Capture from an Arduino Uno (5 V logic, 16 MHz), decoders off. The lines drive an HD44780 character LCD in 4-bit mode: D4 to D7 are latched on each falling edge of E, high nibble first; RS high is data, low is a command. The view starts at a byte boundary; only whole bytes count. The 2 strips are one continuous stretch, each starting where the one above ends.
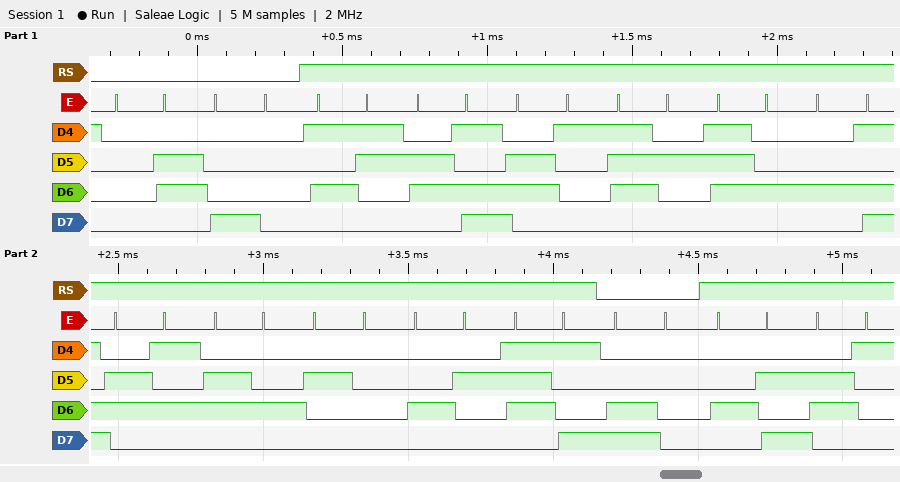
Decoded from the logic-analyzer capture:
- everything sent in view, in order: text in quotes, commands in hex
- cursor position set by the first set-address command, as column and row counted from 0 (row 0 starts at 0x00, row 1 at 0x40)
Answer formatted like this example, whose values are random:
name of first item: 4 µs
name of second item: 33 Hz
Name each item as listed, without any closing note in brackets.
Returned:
everything sent in view, in order: text in quotes, commands in hex: 0x06 0x80 "SmartMed By" 0xC0 "Ja"
cursor position set by the first set-address command, as column and row counted from 0: column 0, row 0
